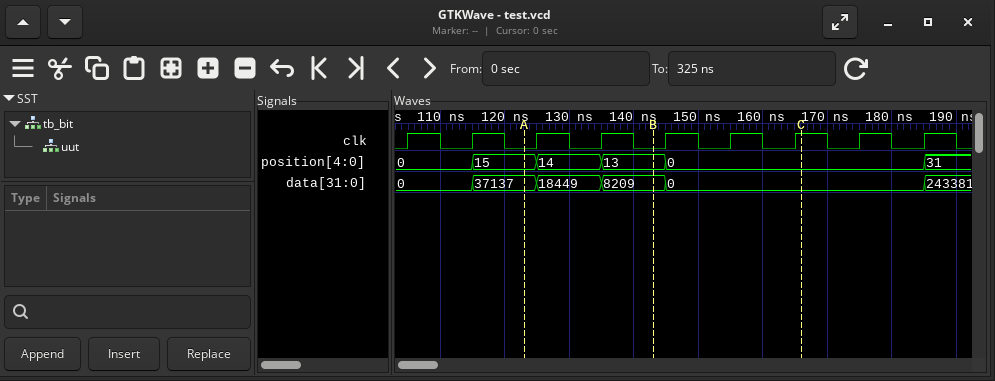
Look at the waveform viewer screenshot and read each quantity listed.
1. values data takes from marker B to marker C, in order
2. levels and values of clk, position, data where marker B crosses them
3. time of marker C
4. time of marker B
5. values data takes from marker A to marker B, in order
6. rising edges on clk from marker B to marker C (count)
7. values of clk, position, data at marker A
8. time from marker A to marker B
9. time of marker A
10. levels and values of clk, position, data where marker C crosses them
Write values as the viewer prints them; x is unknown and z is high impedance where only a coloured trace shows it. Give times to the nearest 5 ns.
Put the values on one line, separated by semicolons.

8209, 0; clk=0, position=13, data=8209; 165 ns; 145 ns; 37137, 18449, 8209; 3; clk=0, position=15, data=37137; 20 ns; 125 ns; clk=1, position=0, data=0
